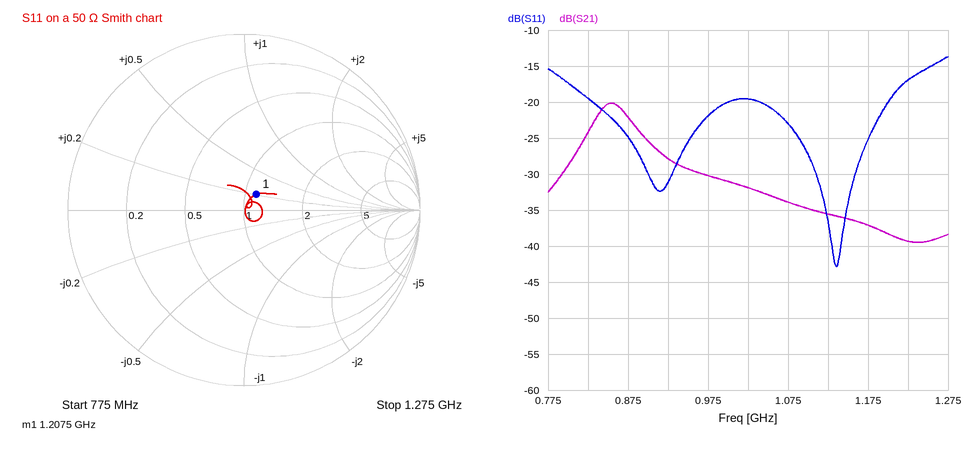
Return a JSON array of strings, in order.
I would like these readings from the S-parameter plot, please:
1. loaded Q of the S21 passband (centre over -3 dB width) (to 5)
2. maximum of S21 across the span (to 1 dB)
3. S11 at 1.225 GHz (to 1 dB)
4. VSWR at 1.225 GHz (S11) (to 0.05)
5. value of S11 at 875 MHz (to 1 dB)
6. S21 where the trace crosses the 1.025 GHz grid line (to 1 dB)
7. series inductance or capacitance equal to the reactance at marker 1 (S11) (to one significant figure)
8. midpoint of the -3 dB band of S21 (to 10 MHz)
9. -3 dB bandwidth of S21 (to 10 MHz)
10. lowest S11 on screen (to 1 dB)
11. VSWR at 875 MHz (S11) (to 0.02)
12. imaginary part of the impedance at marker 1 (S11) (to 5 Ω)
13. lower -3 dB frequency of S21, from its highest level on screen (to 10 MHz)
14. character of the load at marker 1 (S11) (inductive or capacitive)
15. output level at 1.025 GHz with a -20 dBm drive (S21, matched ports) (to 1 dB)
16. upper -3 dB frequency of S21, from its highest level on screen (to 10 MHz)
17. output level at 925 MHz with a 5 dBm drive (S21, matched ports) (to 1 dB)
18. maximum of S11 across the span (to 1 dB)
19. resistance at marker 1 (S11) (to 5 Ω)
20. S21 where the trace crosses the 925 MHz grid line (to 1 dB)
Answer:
["15", "-20 dB", "-17 dB", "1.35", "-25 dB", "-32 dB", "1 nH", "860 MHz", "50 MHz", "-43 dB", "1.12", "+10 Ω", "830 MHz", "inductive", "-52 dBm", "880 MHz", "-23 dBm", "-14 dB", "55 Ω", "-28 dB"]
